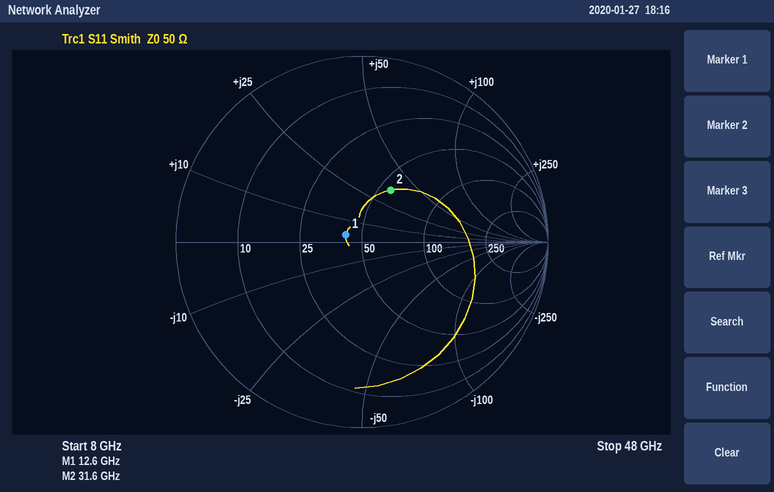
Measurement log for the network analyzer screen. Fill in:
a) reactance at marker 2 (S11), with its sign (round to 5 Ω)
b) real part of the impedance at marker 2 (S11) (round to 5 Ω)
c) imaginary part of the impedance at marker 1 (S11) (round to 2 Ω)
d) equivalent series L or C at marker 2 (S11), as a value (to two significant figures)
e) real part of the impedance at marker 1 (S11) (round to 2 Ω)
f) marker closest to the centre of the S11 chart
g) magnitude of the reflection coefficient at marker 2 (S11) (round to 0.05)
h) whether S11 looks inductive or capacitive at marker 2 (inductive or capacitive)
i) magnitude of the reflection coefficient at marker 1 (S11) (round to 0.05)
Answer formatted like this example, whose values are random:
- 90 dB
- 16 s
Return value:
- +35 Ω
- 55 Ω
- +4 Ω
- 180 pH
- 42 Ω
- marker 1
- 0.30
- inductive
- 0.10
